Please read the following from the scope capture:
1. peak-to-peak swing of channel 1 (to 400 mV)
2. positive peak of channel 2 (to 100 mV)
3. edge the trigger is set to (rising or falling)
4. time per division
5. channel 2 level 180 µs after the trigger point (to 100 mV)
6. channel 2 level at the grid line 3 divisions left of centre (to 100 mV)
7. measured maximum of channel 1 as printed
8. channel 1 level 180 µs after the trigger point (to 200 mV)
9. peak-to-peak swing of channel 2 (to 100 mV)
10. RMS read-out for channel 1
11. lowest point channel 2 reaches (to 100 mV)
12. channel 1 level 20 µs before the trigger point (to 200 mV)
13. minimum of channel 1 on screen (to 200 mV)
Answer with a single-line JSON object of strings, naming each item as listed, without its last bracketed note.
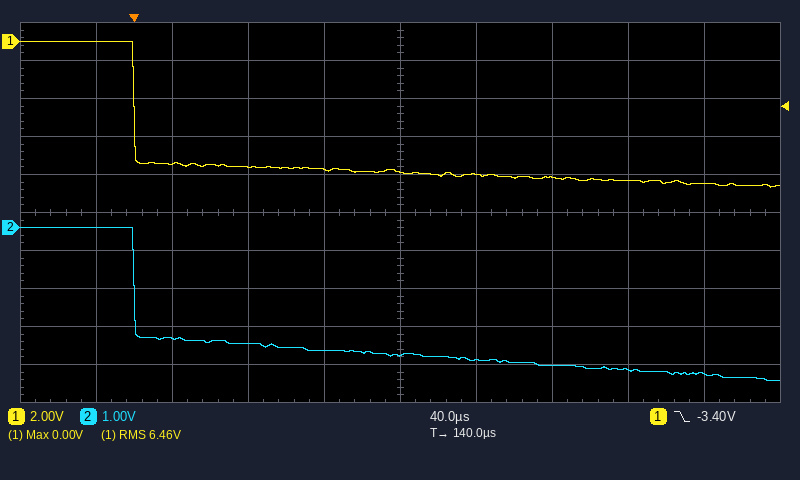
{"peak-to-peak swing of channel 1": "7.6 V", "positive peak of channel 2": "0.0 V", "edge the trigger is set to": "falling", "time per division": "40 µs", "channel 2 level 180 µs after the trigger point": "-3.5 V", "channel 2 level at the grid line 3 divisions left of centre": "-2.9 V", "measured maximum of channel 1 as printed": "0.00 V", "channel 1 level 180 µs after the trigger point": "-7.0 V", "peak-to-peak swing of channel 2": "4.0 V", "RMS read-out for channel 1": "6.46 V", "lowest point channel 2 reaches": "-4.0 V", "channel 1 level 20 µs before the trigger point": "0.0 V", "minimum of channel 1 on screen": "-7.6 V"}
